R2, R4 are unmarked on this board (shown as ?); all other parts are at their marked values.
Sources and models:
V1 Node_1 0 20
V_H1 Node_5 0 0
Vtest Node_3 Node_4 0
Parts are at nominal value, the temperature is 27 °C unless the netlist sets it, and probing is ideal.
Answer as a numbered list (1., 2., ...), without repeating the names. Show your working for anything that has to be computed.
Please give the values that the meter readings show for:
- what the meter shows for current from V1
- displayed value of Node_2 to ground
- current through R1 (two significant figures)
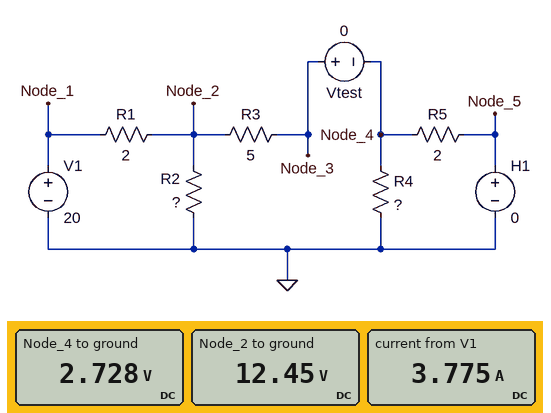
1. 3.775 A
2. 12.45 V
3. (20 V - 12.45 V) / 2 Ω = 3.8 A
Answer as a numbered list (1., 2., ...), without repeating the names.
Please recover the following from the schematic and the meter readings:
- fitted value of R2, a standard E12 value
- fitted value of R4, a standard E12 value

1. 6.8 Ω
2. 4.7 Ω
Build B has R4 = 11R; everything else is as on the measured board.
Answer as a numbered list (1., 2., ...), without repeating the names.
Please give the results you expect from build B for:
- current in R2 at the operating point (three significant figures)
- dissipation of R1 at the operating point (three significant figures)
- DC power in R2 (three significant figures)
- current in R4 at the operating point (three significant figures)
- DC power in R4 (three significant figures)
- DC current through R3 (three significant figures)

1. 1.85 A
2. 27.7 W
3. 23.2 W
4. 289 mA
5. 916 mW
6. 1.88 A
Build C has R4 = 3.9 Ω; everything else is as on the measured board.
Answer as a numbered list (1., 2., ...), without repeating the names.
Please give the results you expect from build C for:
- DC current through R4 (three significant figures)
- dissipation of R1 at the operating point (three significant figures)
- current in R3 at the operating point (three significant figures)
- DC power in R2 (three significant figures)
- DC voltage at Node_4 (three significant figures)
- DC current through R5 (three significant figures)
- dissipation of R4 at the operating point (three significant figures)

1. 666 mA
2. 28.7 W
3. 1.96 A
4. 22.7 W
5. 2.60 V
6. 1.30 A
7. 1.73 W
